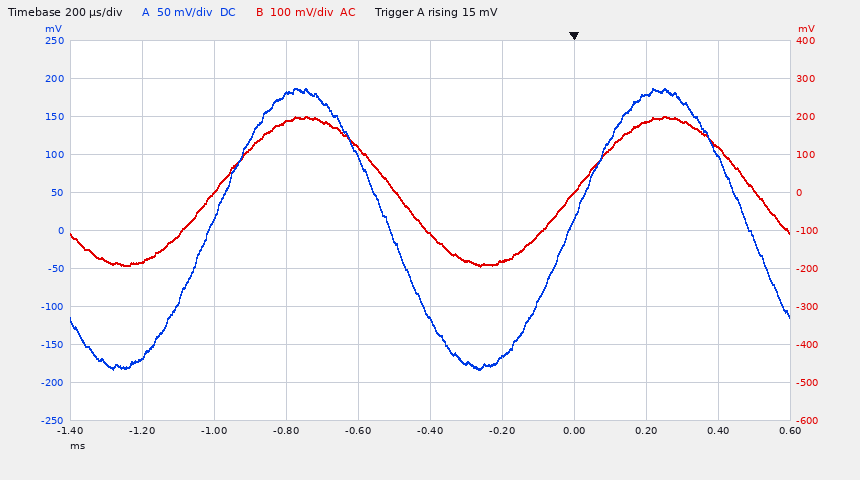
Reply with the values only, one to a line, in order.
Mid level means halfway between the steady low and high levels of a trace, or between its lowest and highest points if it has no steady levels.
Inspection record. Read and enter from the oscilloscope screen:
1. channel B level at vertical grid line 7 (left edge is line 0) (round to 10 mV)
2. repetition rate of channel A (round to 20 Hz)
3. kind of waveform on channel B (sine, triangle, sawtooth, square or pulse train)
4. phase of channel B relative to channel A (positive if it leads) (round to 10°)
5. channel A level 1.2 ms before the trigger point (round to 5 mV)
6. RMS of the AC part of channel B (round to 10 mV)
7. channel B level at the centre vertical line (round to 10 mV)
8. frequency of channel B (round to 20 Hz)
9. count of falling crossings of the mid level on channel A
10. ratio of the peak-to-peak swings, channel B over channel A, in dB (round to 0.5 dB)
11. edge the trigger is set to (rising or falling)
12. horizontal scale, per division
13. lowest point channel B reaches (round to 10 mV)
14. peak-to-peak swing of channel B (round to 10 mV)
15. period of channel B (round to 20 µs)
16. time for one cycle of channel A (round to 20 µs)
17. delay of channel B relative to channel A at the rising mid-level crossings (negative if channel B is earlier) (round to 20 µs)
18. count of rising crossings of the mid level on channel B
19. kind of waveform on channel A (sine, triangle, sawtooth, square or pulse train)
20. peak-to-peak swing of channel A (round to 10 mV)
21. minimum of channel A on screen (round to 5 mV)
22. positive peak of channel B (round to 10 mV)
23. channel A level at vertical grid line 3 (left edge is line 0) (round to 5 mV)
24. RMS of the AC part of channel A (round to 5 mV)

0 mV
1.00 kHz
sine
-10°
-165 mV
140 mV
-110 mV
1.00 kHz
2
0.5 dB
rising
200 µs
-190 mV
390 mV
1.00 ms
1.00 ms
+20 µs
2
sine
370 mV
-185 mV
200 mV
180 mV
130 mV
